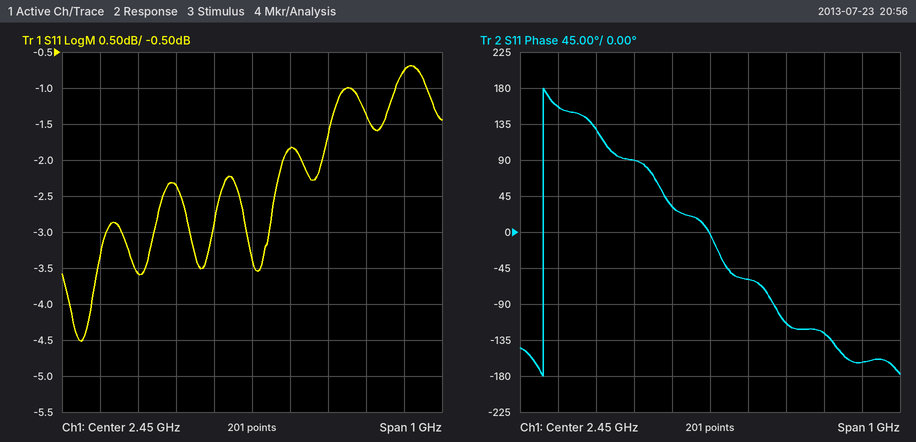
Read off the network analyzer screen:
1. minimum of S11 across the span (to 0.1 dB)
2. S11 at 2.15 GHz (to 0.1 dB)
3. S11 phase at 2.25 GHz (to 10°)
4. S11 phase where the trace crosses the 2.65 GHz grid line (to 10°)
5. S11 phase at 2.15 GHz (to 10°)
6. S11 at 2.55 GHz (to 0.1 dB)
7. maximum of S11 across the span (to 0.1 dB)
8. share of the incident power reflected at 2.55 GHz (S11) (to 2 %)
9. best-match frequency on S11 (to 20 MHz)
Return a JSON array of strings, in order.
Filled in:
["-4.5 dB", "-3.6 dB", "90°", "-110°", "130°", "-1.8 dB", "-0.7 dB", "66 %", "2.00 GHz"]
